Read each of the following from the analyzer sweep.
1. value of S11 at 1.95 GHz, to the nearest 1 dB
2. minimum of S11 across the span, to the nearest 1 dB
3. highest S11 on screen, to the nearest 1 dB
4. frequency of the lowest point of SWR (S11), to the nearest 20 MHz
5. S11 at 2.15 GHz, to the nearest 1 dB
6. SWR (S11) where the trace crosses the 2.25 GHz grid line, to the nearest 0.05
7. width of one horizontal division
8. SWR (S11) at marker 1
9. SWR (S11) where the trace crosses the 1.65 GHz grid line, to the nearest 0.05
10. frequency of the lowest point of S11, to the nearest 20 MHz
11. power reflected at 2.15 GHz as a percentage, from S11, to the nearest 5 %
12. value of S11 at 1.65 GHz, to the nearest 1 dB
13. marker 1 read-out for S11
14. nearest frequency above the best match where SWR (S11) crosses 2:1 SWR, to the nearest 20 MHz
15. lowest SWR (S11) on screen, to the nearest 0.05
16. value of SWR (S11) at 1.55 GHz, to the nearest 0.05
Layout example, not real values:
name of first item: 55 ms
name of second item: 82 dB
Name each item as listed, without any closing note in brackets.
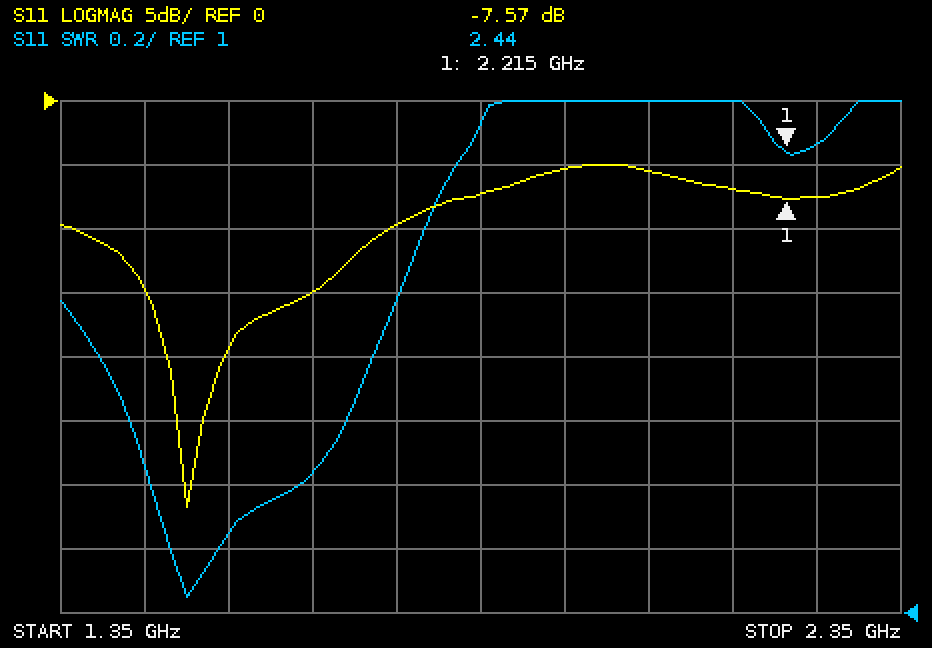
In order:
value of S11 at 1.95 GHz, to the nearest 1 dB: -5 dB
minimum of S11 across the span, to the nearest 1 dB: -32 dB
highest S11 on screen, to the nearest 1 dB: -5 dB
frequency of the lowest point of SWR (S11), to the nearest 20 MHz: 1.50 GHz
S11 at 2.15 GHz, to the nearest 1 dB: -7 dB
SWR (S11) where the trace crosses the 2.25 GHz grid line, to the nearest 0.05: 2.45
width of one horizontal division: 100 MHz
SWR (S11) at marker 1: 2.44
SWR (S11) where the trace crosses the 1.65 GHz grid line, to the nearest 0.05: 1.45
frequency of the lowest point of S11, to the nearest 20 MHz: 1.50 GHz
power reflected at 2.15 GHz as a percentage, from S11, to the nearest 5 %: 20 %
value of S11 at 1.65 GHz, to the nearest 1 dB: -15 dB
marker 1 read-out for S11: -7.57 dB
nearest frequency above the best match where SWR (S11) crosses 2:1 SWR, to the nearest 20 MHz: 1.76 GHz
lowest SWR (S11) on screen, to the nearest 0.05: 1.05
value of SWR (S11) at 1.55 GHz, to the nearest 0.05: 1.25
